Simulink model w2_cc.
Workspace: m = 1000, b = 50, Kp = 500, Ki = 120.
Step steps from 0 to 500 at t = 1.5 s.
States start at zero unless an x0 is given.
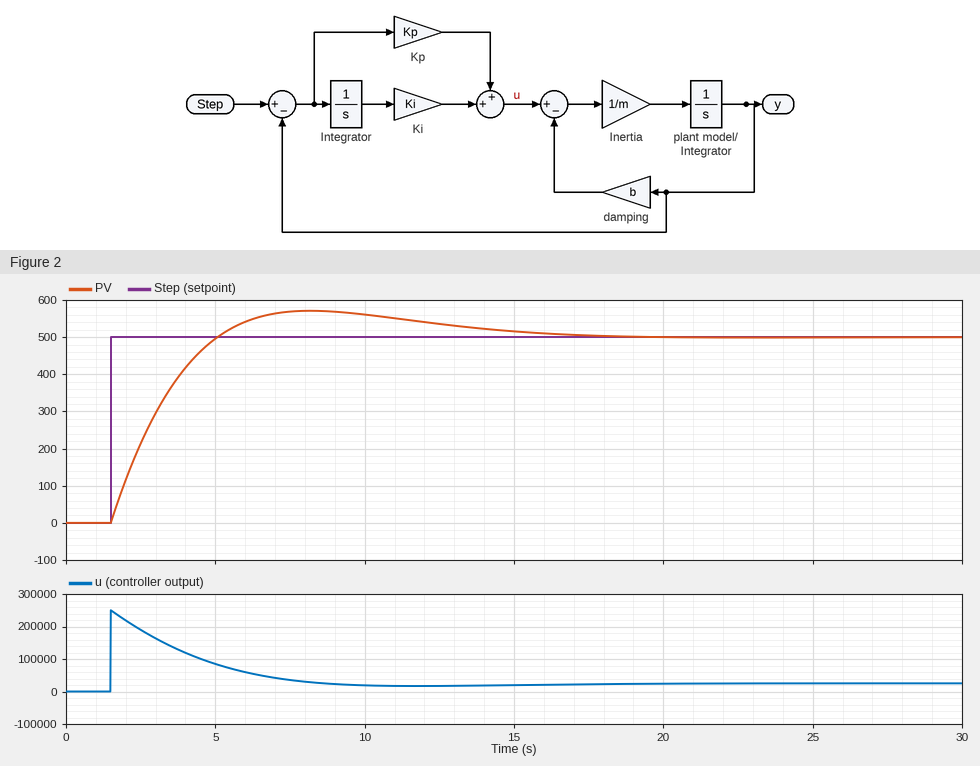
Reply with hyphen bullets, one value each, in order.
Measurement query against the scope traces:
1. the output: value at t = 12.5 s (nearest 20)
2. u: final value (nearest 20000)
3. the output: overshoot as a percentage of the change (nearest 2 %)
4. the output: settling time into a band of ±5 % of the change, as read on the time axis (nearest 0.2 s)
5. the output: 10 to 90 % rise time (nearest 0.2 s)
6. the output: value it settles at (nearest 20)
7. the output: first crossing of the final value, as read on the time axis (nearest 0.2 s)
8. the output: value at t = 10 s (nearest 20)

- 540
- 20000
- 14 %
- 13.6 s
- 2.6 s
- 500
- 5.0 s
- 560
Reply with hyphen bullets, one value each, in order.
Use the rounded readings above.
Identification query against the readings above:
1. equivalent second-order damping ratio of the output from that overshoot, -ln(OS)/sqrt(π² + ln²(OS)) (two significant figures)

- 0.53
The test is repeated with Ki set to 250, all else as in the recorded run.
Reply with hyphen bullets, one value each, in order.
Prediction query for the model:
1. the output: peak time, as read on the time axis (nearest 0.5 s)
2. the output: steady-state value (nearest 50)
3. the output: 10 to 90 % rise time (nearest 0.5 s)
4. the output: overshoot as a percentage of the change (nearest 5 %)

- 6.5 s
- 500
- 2.0 s
- 25 %
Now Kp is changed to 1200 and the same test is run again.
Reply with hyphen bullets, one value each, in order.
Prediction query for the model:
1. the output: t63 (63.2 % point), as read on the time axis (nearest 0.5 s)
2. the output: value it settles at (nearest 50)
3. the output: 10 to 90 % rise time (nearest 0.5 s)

- 2.5 s
- 500
- 1.5 s
